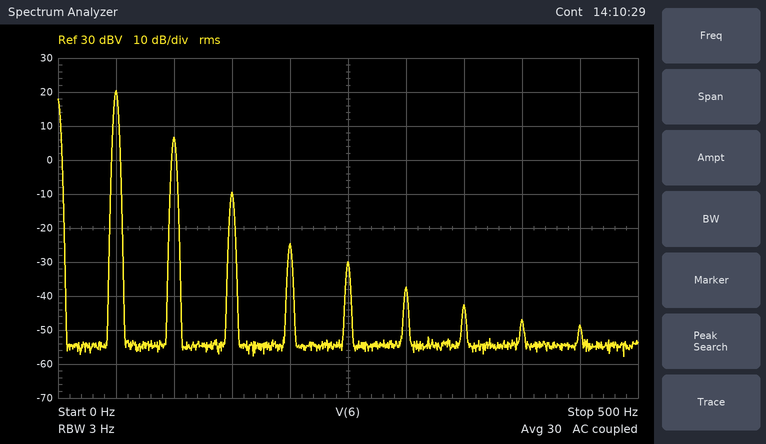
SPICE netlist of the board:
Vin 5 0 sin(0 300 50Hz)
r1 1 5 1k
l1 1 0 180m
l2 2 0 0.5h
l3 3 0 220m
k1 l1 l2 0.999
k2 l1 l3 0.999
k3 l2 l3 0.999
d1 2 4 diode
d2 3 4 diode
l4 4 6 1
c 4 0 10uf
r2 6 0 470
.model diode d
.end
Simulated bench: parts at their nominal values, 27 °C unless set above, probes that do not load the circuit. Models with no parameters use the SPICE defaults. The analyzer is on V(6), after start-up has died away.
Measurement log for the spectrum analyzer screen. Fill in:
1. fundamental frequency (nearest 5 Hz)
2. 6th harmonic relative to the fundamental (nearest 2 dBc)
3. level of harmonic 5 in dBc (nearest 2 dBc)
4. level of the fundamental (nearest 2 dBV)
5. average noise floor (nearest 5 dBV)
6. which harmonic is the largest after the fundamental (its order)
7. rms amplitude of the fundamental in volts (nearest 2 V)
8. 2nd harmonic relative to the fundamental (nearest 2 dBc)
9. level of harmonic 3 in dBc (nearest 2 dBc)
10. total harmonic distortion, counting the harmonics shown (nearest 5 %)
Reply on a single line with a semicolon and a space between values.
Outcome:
50 Hz; -58 dBc; -50 dBc; 20 dBV; -55 dBV; 2; 10 V; -14 dBc; -30 dBc; 20 %
